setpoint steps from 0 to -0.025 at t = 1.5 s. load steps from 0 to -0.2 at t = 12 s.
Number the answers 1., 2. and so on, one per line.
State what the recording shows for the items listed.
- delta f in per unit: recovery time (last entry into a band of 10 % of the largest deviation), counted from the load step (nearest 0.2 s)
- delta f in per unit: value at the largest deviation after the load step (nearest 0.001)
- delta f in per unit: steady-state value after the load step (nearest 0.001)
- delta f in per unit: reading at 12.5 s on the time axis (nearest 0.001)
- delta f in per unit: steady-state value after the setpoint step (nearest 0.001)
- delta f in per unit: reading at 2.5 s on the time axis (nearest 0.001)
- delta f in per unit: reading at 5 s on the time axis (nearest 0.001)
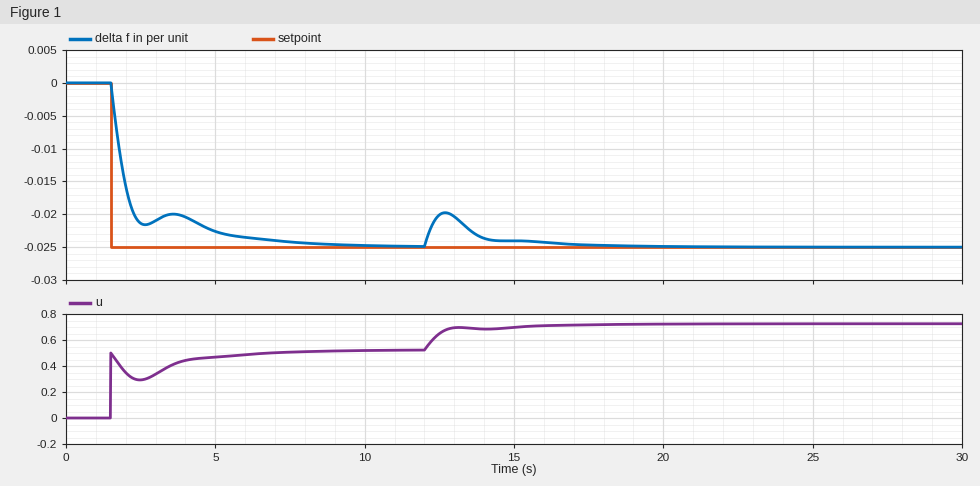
1. 4.6 s
2. -0.020
3. -0.025
4. -0.020
5. -0.025
6. -0.021
7. -0.023
